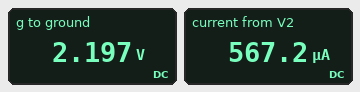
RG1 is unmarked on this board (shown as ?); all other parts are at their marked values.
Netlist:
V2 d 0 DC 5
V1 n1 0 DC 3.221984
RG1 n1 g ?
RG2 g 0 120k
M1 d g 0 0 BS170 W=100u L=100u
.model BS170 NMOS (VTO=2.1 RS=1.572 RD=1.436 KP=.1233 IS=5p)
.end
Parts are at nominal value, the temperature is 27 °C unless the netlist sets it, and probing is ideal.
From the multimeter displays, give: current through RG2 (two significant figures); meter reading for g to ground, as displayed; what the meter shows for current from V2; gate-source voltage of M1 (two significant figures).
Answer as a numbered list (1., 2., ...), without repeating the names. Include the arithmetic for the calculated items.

1. (2.197 V) / 120 kΩ = 18 µA
2. 2.197 V
3. 567.2 µA
4. 2.197 V = 2.2 V
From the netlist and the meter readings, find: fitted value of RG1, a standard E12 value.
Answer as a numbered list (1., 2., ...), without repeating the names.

1. 56 kΩ
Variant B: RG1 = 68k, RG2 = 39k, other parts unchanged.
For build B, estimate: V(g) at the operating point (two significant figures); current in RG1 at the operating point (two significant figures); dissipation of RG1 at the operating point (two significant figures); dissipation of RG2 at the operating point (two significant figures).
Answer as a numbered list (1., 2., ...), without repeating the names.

1. 1.2 V
2. 30 µA
3. 62 µW
4. 35 µW
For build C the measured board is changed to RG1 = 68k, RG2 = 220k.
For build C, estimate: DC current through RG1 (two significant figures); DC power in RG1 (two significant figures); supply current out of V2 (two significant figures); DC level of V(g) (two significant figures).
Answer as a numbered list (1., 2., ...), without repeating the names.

1. 11 µA
2. 8.5 µW
3. 7.5 mA
4. 2.5 V
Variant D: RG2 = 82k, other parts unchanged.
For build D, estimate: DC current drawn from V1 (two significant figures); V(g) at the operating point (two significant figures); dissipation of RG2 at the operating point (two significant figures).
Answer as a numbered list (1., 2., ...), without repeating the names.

1. 23 µA
2. 1.9 V
3. 45 µW
